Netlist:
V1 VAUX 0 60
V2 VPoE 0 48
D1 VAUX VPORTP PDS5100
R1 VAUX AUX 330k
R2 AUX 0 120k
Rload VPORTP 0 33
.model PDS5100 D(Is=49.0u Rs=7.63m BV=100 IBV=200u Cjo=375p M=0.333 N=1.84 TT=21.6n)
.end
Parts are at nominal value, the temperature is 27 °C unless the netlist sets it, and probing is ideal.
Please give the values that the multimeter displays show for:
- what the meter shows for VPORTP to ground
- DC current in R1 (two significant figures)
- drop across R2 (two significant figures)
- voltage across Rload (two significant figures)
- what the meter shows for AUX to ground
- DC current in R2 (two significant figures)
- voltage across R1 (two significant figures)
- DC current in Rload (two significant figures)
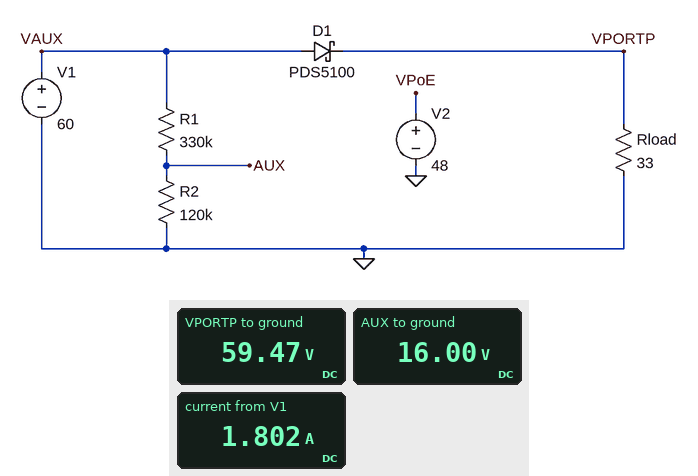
59.47 V
130 µA
16 V
59 V
16.00 V
130 µA
44 V
1.8 A
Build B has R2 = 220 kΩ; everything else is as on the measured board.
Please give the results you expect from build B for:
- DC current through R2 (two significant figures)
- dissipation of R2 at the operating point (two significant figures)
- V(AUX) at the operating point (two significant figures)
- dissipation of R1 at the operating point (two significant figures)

110 µA
2.6 mW
24 V
3.9 mW
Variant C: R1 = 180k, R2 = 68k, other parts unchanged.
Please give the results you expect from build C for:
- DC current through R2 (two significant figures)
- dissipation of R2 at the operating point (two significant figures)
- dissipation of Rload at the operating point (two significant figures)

240 µA
4.0 mW
110 W
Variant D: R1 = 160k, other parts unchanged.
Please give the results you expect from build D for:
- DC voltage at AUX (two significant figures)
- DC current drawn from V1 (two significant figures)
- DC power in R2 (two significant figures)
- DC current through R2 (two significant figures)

26 V
1.8 A
5.5 mW
210 µA
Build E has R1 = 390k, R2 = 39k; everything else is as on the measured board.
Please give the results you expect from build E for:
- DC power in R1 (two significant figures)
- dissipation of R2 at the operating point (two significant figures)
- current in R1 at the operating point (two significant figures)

7.6 mW
760 µW
140 µA
